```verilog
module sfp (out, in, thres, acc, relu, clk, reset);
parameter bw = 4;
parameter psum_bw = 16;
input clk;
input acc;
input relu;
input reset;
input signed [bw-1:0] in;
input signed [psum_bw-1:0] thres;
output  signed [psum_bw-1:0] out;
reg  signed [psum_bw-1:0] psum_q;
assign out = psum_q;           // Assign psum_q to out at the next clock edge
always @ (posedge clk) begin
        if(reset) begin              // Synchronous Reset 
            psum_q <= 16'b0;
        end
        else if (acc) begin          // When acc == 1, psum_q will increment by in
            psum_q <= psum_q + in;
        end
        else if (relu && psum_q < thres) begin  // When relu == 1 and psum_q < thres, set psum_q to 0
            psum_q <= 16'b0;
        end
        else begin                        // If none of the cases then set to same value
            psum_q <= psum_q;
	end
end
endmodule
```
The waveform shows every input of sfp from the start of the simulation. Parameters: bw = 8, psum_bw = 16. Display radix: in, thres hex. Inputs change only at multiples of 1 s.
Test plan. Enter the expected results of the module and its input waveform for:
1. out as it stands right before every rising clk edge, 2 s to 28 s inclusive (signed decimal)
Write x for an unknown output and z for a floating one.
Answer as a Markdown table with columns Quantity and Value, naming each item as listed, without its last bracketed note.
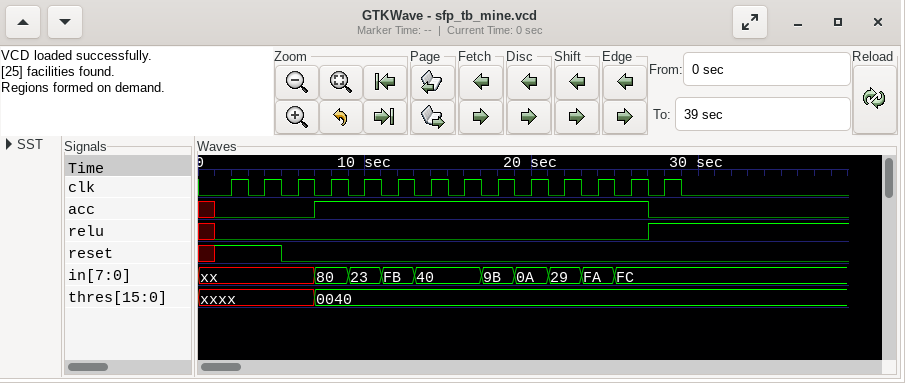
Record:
| Quantity | Value |
|---|---|
| out as it stands right before every rising clk edge, 2 s to 28 s inclusive | x, 0, 0, 0, -128, -93, -98, -34, 30, -71, -61, -20, -26, -30 |
